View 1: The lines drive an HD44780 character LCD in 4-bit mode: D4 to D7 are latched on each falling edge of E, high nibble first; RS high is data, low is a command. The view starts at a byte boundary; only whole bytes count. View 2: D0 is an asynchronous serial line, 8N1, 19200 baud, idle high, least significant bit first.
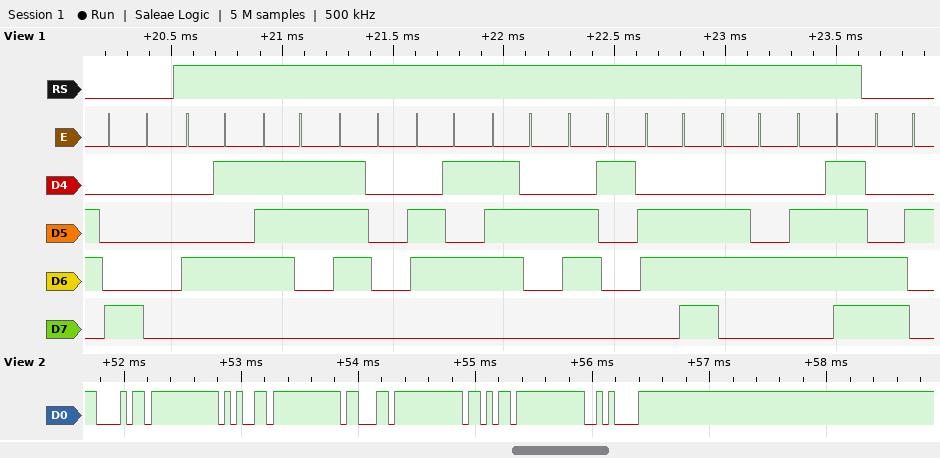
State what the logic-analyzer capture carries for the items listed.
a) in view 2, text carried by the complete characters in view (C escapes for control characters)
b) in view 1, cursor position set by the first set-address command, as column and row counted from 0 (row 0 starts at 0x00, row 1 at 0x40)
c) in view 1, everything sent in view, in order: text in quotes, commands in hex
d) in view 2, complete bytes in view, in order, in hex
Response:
"heck\n"
column 0, row 0
0x80 "Esperando" 0xC2
0x68 0x65 0x63 0x6B 0x0A
